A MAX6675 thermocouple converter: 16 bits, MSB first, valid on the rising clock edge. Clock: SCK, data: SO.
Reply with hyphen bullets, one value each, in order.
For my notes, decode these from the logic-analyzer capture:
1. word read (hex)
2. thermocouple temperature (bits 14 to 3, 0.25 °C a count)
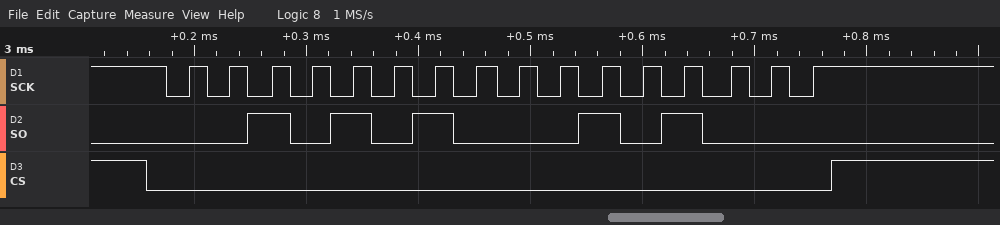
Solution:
- 0x2A28
- 337.25 °C
